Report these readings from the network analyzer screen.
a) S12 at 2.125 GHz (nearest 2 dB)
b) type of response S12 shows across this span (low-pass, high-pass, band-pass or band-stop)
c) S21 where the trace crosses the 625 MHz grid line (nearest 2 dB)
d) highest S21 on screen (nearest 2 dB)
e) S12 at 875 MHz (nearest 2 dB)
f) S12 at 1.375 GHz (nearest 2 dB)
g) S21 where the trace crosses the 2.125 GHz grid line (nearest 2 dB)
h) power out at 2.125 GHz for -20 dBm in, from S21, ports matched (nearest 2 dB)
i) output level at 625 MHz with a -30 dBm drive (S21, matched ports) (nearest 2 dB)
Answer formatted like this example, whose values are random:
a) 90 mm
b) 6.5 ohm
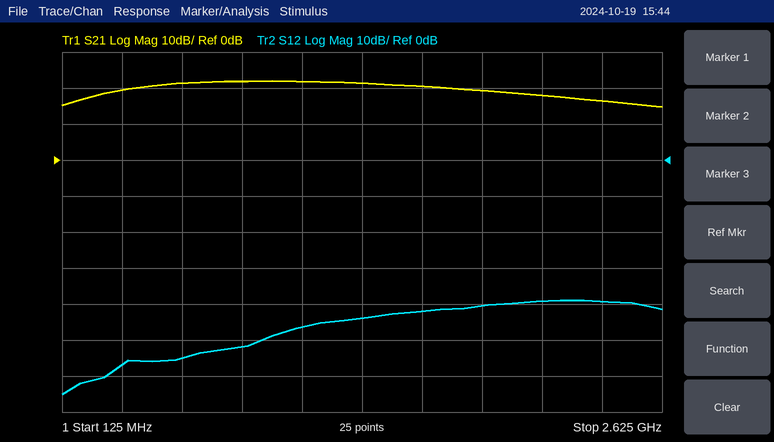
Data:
a) -40 dB
b) high-pass
c) 22 dB
d) 22 dB
e) -52 dB
f) -44 dB
g) 18 dB
h) -2 dBm
i) -8 dBm
